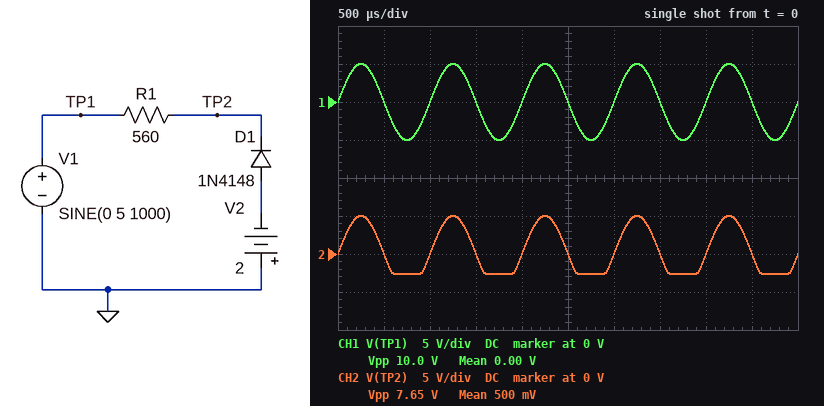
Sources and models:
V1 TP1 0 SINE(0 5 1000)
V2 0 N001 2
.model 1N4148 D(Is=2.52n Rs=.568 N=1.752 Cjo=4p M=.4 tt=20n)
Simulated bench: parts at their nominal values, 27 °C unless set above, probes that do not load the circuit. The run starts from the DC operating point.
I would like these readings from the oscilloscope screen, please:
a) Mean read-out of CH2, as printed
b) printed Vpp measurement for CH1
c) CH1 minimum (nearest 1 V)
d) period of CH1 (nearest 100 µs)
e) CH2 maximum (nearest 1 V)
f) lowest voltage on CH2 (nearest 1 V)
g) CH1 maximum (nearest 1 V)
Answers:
500 mV
10.0 V
-5 V
1.0 ms
5 V
-3 V
5 V
